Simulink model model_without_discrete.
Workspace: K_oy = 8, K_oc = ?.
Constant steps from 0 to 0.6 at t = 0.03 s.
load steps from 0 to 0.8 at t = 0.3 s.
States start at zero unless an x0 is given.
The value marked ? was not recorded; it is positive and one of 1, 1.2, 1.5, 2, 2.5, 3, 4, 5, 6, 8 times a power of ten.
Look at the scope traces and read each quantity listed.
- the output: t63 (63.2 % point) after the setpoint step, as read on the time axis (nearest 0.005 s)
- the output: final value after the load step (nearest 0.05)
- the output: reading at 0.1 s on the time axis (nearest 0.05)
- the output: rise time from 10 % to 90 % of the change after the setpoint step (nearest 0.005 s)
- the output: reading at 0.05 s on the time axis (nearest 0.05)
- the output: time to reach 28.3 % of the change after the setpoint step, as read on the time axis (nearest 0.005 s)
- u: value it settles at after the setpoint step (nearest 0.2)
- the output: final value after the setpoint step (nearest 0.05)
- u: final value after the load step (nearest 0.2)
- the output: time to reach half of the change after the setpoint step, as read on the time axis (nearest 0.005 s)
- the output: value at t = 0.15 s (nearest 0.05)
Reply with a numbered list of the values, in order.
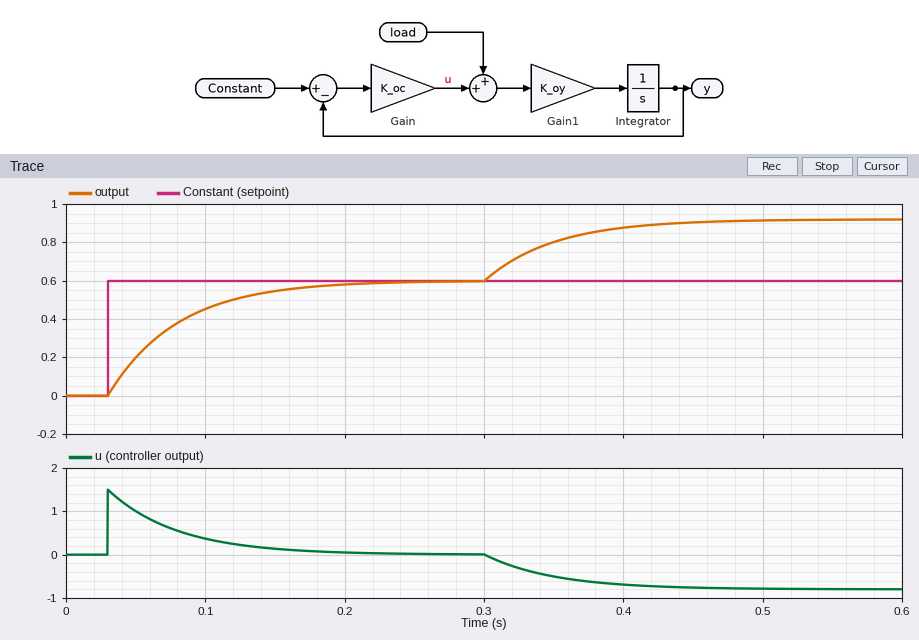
1. 0.080 s
2. 0.90
3. 0.45
4. 0.110 s
5. 0.20
6. 0.045 s
7. 0.0
8. 0.60
9. -0.8
10. 0.065 s
11. 0.55
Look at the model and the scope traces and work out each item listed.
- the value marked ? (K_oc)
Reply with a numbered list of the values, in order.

1. 2.5
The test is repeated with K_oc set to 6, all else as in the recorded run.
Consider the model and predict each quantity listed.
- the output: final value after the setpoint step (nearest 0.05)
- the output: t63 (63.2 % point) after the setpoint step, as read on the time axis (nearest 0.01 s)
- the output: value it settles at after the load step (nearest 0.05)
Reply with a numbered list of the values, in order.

1. 0.60
2. 0.05 s
3. 0.75
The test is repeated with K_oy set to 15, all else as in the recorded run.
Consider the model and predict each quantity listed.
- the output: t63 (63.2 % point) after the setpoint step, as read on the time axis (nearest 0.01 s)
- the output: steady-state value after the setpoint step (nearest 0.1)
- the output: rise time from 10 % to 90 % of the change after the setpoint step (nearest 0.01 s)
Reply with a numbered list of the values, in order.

1. 0.06 s
2. 0.6
3. 0.06 s
